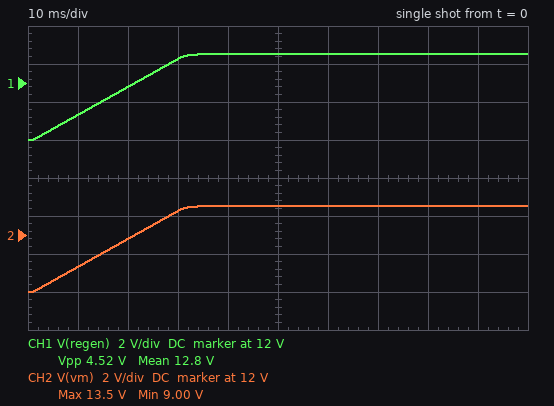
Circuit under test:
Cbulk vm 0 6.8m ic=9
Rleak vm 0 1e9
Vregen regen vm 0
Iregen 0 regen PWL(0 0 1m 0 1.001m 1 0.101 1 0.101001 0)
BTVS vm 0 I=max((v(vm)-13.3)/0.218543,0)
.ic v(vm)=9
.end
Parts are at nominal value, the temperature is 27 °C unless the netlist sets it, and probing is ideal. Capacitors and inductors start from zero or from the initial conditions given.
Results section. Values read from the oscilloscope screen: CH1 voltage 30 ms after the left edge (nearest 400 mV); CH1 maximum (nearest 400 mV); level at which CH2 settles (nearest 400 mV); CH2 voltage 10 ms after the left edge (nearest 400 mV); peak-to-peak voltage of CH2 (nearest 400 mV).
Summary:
13.2 V
13.6 V
13.6 V
10.4 V
4.4 V
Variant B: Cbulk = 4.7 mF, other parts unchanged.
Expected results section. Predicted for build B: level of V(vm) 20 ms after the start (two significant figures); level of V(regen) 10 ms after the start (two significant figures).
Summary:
13 V
11 V
